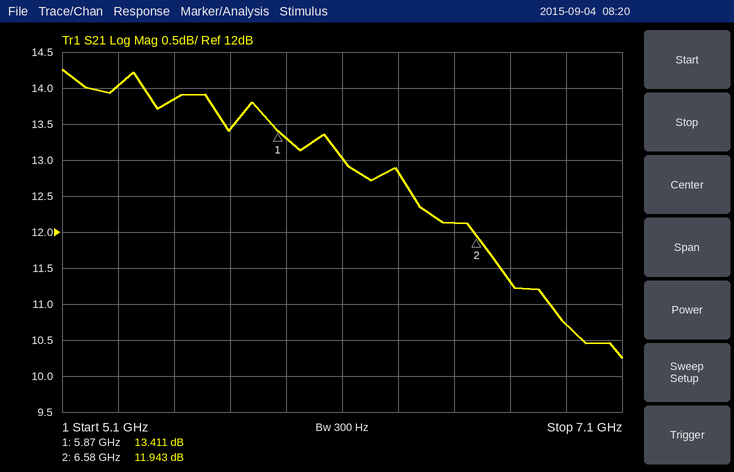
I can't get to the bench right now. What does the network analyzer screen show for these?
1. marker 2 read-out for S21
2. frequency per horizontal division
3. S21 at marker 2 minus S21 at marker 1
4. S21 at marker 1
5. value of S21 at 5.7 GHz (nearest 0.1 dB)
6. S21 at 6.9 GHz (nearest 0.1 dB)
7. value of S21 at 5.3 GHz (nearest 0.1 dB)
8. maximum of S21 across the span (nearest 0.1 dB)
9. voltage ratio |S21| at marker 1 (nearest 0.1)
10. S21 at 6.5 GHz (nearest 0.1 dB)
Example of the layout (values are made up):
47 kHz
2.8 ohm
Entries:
11.943 dB
200 MHz
-1.468 dB
13.411 dB
13.4 dB
10.7 dB
14.0 dB
14.3 dB
4.7
12.1 dB
